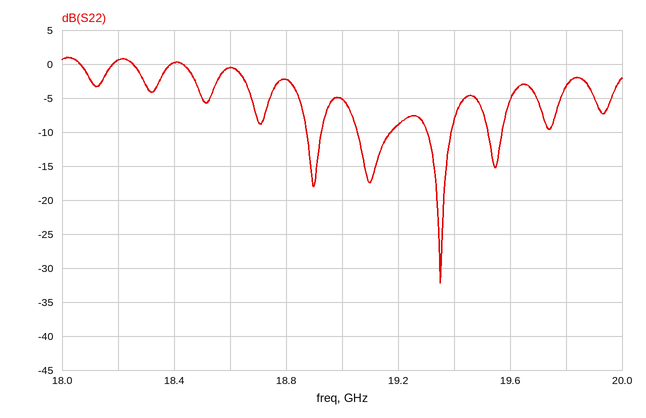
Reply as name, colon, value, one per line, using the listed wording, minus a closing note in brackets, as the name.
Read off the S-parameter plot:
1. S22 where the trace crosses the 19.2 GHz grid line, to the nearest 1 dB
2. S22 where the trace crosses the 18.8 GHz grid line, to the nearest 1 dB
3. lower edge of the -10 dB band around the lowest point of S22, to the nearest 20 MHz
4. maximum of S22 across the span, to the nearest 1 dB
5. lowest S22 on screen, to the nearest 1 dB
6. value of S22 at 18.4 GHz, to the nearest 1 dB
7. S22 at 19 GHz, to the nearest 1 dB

S22 where the trace crosses the 19.2 GHz grid line, to the nearest 1 dB: -9 dB
S22 where the trace crosses the 18.8 GHz grid line, to the nearest 1 dB: -2 dB
lower edge of the -10 dB band around the lowest point of S22, to the nearest 20 MHz: 19.30 GHz
maximum of S22 across the span, to the nearest 1 dB: 1 dB
lowest S22 on screen, to the nearest 1 dB: -32 dB
value of S22 at 18.4 GHz, to the nearest 1 dB: 0 dB
S22 at 19 GHz, to the nearest 1 dB: -5 dB
